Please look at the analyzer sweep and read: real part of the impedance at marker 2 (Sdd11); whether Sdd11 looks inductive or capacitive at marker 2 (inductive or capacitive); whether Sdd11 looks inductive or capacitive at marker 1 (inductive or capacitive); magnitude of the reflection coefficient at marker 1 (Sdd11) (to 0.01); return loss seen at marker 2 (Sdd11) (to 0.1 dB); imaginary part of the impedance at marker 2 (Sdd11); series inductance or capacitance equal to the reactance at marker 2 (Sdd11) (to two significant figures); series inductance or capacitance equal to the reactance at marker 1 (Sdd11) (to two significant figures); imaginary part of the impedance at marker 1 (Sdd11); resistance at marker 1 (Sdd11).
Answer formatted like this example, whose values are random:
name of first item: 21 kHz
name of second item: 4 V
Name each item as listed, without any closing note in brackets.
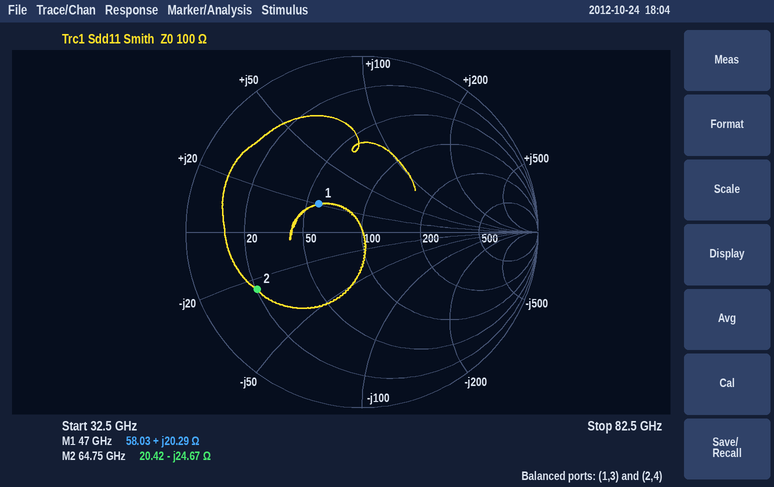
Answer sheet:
real part of the impedance at marker 2: 20.42 Ω
whether Sdd11 looks inductive or capacitive at marker 2: capacitive
whether Sdd11 looks inductive or capacitive at marker 1: inductive
magnitude of the reflection coefficient at marker 1 (Sdd11): 0.29
return loss seen at marker 2 (Sdd11): 3.4 dB
imaginary part of the impedance at marker 2: -24.67 Ω
series inductance or capacitance equal to the reactance at marker 2 (Sdd11): 100 fF
series inductance or capacitance equal to the reactance at marker 1 (Sdd11): 69 pH
imaginary part of the impedance at marker 1: +20.29 Ω
resistance at marker 1: 58.03 Ω
